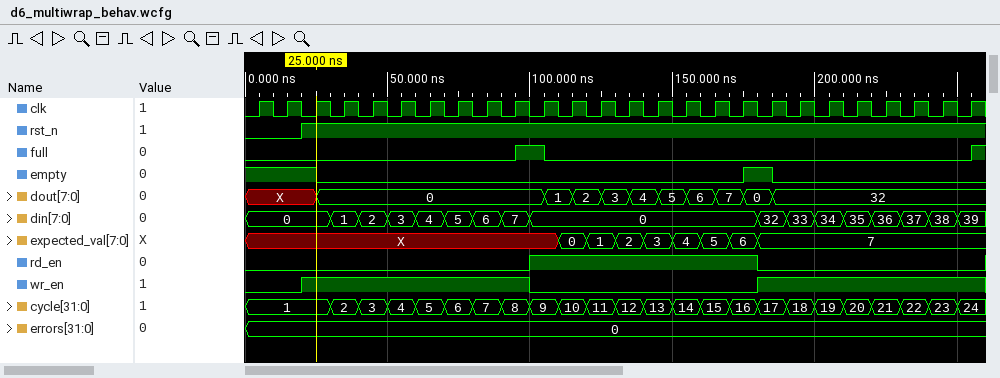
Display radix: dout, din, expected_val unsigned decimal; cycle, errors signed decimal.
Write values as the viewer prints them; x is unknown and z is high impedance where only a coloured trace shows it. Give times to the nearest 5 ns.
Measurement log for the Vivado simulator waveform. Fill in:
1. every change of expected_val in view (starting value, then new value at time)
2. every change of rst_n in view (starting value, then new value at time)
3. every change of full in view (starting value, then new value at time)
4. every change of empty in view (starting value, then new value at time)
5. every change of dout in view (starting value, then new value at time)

X, 0 at 110 ns, 1 at 120 ns, 2 at 130 ns, 3 at 140 ns, 4 at 150 ns, 5 at 160 ns, 6 at 170 ns, 7 at 180 ns
0, 1 at 20 ns
0, 1 at 95 ns, 0 at 105 ns, 1 at 255 ns
1, 0 at 25 ns, 1 at 175 ns, 0 at 185 ns
X, 0 at 25 ns, 1 at 105 ns, 2 at 115 ns, 3 at 125 ns, 4 at 135 ns, 5 at 145 ns, 6 at 155 ns, 7 at 165 ns, 0 at 175 ns, 32 at 185 ns
